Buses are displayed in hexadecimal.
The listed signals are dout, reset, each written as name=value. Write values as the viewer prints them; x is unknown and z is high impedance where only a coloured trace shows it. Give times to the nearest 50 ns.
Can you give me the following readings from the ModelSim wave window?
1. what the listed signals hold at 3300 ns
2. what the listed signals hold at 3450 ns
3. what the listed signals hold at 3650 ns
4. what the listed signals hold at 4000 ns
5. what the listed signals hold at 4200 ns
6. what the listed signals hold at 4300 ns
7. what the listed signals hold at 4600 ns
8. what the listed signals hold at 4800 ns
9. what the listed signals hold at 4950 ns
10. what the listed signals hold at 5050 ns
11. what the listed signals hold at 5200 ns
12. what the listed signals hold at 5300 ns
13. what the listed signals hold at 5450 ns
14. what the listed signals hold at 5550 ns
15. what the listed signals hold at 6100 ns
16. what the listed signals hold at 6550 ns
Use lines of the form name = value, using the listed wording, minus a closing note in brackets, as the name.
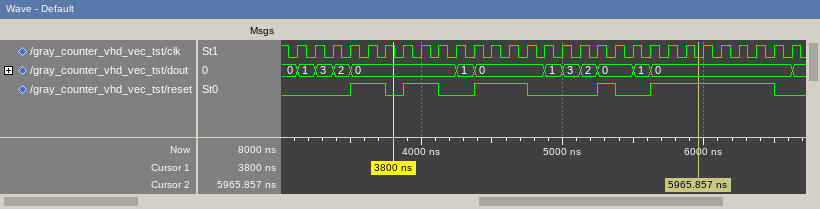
what the listed signals hold at 3300 ns = dout=3, reset=0
what the listed signals hold at 3450 ns = dout=2, reset=0
what the listed signals hold at 3650 ns = dout=0, reset=1
what the listed signals hold at 4000 ns = dout=0, reset=1
what the listed signals hold at 4200 ns = dout=0, reset=0
what the listed signals hold at 4300 ns = dout=1, reset=0
what the listed signals hold at 4600 ns = dout=0, reset=1
what the listed signals hold at 4800 ns = dout=0, reset=0
what the listed signals hold at 4950 ns = dout=1, reset=0
what the listed signals hold at 5050 ns = dout=3, reset=0
what the listed signals hold at 5200 ns = dout=2, reset=0
what the listed signals hold at 5300 ns = dout=0, reset=1
what the listed signals hold at 5450 ns = dout=0, reset=0
what the listed signals hold at 5550 ns = dout=1, reset=0
what the listed signals hold at 6100 ns = dout=0, reset=1
what the listed signals hold at 6550 ns = dout=0, reset=0
